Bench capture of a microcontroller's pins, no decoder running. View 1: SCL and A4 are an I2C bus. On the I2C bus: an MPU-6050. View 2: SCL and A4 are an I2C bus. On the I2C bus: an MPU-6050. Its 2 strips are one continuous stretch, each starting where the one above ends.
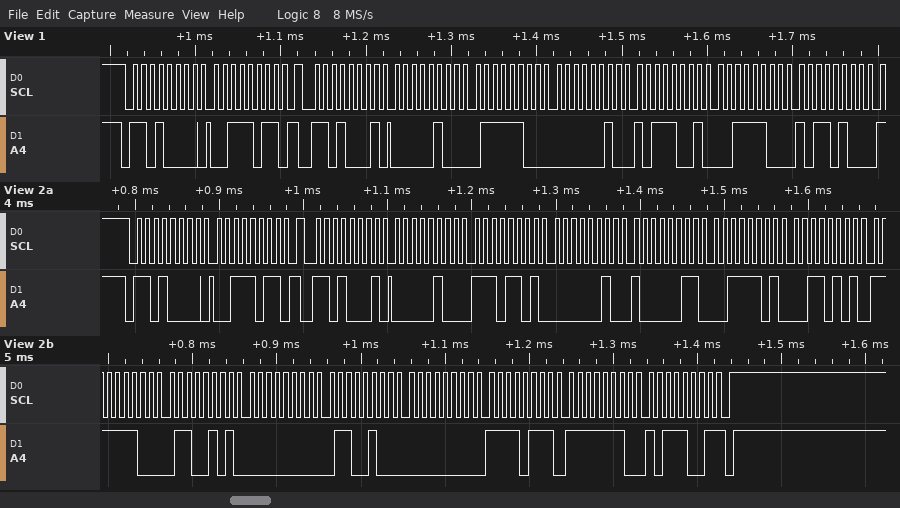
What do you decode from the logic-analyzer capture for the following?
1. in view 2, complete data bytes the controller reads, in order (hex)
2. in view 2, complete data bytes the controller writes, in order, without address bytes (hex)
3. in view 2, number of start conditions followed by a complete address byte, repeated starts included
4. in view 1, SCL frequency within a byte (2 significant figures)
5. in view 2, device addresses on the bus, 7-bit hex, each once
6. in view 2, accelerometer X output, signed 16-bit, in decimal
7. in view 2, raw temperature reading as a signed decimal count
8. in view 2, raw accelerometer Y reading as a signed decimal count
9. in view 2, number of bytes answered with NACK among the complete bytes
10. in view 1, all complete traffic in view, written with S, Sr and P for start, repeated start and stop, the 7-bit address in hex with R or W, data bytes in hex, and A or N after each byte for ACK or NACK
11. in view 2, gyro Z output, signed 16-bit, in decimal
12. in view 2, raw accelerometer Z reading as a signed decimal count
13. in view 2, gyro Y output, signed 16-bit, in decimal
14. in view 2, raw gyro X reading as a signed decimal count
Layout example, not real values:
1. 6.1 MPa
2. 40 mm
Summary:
1. 04 ED 02 83 3D 35 FC 65 00 64 00 F7 FE B9
2. 3B
3. 2
4. 100 kHz
5. 0x68
6. 1261
7. -923
8. 643
9. 1
10. S 68W A 3B A Sr 68R A 04 A 7C A 02 A B9 A 3C A B4 A
11. -327
12. 15669
13. 247
14. 100
